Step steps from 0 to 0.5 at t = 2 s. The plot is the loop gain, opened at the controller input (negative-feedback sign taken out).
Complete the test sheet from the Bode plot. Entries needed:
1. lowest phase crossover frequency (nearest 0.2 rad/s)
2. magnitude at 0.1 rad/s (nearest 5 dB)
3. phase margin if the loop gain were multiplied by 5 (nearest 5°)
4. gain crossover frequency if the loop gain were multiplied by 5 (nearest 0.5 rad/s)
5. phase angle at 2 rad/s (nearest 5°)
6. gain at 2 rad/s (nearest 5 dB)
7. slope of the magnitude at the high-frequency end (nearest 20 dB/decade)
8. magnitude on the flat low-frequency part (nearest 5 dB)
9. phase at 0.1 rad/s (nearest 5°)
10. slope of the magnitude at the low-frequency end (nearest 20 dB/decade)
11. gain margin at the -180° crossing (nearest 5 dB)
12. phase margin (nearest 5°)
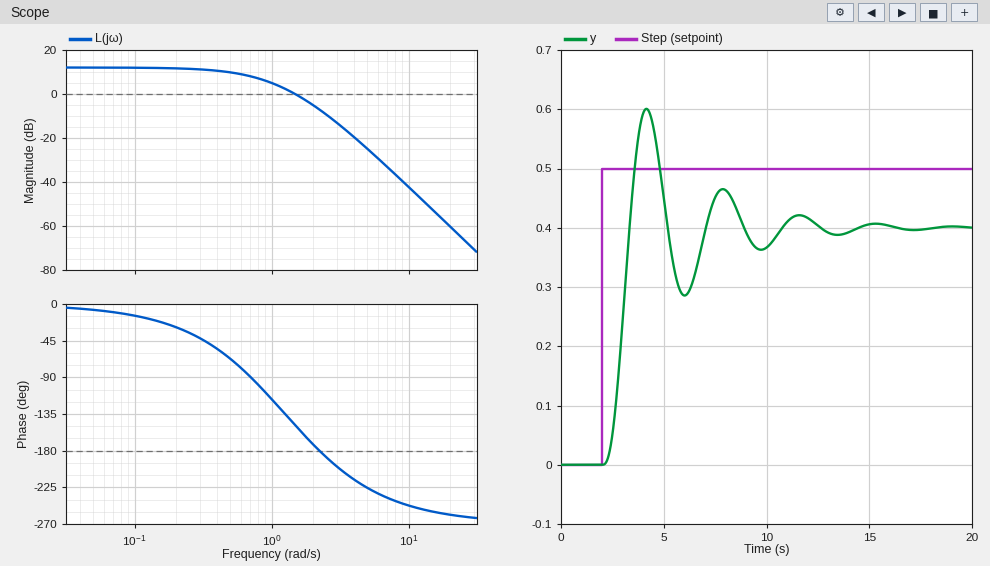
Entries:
2.2 rad/s
10 dB
-20°
3.0 rad/s
-170°
-5 dB
-60 dB/decade
10 dB
-15°
0 dB/decade
5 dB
30°
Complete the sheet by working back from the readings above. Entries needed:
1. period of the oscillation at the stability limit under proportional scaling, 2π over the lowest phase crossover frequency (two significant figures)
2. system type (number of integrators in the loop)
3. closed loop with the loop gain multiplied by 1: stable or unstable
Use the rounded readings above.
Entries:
2.9 s
0
stable
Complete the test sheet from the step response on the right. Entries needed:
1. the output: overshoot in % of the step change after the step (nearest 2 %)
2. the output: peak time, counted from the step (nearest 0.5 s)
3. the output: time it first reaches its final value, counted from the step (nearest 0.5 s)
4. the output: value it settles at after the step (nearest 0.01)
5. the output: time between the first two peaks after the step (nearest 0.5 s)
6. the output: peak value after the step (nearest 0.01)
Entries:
50 %
2.0 s
1.5 s
0.40
3.5 s
0.60
